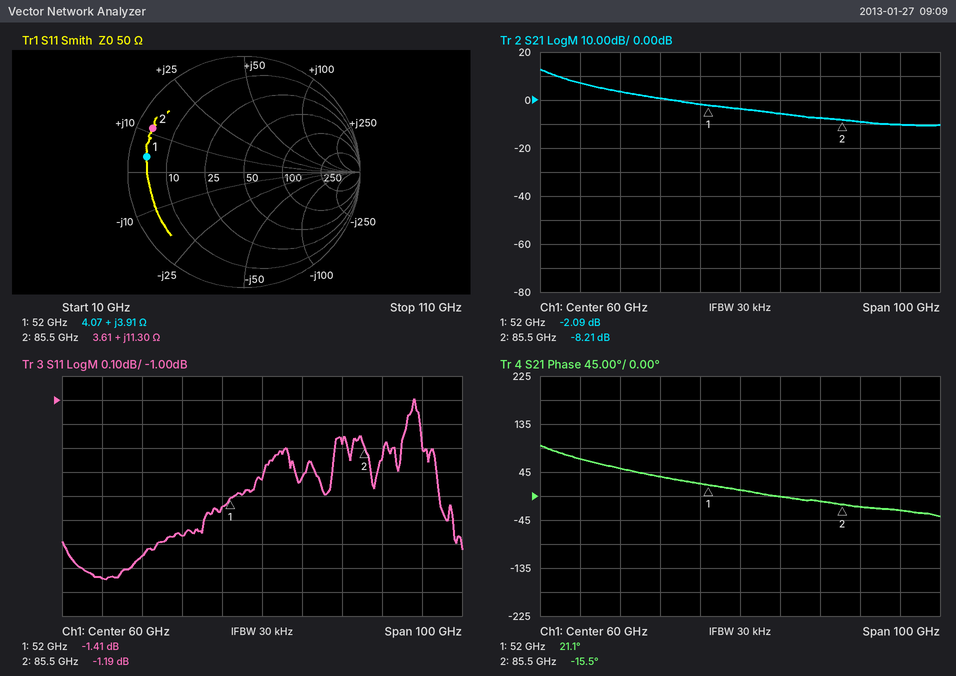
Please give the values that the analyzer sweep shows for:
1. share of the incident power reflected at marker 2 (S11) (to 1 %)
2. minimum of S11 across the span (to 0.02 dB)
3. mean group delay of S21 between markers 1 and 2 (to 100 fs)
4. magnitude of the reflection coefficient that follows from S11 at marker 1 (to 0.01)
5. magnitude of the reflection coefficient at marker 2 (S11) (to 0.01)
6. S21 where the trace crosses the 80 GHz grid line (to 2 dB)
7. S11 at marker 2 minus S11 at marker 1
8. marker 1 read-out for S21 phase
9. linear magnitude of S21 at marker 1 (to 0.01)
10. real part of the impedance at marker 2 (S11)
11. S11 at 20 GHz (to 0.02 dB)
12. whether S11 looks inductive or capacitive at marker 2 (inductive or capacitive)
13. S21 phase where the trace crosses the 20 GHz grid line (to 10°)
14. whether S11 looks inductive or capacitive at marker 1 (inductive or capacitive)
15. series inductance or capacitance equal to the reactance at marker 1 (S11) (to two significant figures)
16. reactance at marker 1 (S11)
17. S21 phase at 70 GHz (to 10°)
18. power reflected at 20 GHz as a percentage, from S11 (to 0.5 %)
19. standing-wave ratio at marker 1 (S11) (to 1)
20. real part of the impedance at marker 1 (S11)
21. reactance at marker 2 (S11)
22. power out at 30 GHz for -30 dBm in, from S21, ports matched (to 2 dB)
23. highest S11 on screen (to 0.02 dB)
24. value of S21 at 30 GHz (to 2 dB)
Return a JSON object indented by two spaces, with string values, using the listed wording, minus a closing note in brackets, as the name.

{
  "share of the incident power reflected at marker 2 (S11)": "76 %",
  "minimum of S11 across the span": "-1.74 dB",
  "mean group delay of S21 between markers 1 and 2": "3.0 ps",
  "magnitude of the reflection coefficient that follows from S11 at marker 1": "0.85",
  "magnitude of the reflection coefficient at marker 2 (S11)": "0.87",
  "S21 where the trace crosses the 80 GHz grid line": "-8 dB",
  "S11 at marker 2 minus S11 at marker 1": "0.22 dB",
  "marker 1 read-out for S21 phase": "21.1°",
  "linear magnitude of S21 at marker 1": "0.79",
  "real part of the impedance at marker 2": "3.61 Ω",
  "S11 at 20 GHz": "-1.74 dB",
  "whether S11 looks inductive or capacitive at marker 2": "inductive",
  "S21 phase where the trace crosses the 20 GHz grid line": "70°",
  "whether S11 looks inductive or capacitive at marker 1": "inductive",
  "series inductance or capacitance equal to the reactance at marker 1 (S11)": "12 pH",
  "reactance at marker 1": "+3.91 Ω",
  "S21 phase at 70 GHz": "0°",
  "power reflected at 20 GHz as a percentage, from S11": "67.0 %",
  "standing-wave ratio at marker 1 (S11)": "12",
  "real part of the impedance at marker 1": "4.07 Ω",
  "reactance at marker 2": "+11.30 Ω",
  "power out at 30 GHz for -30 dBm in, from S21, ports matched": "-26 dBm",
  "highest S11 on screen": "-1.00 dB",
  "value of S21 at 30 GHz": "4 dB"
}
